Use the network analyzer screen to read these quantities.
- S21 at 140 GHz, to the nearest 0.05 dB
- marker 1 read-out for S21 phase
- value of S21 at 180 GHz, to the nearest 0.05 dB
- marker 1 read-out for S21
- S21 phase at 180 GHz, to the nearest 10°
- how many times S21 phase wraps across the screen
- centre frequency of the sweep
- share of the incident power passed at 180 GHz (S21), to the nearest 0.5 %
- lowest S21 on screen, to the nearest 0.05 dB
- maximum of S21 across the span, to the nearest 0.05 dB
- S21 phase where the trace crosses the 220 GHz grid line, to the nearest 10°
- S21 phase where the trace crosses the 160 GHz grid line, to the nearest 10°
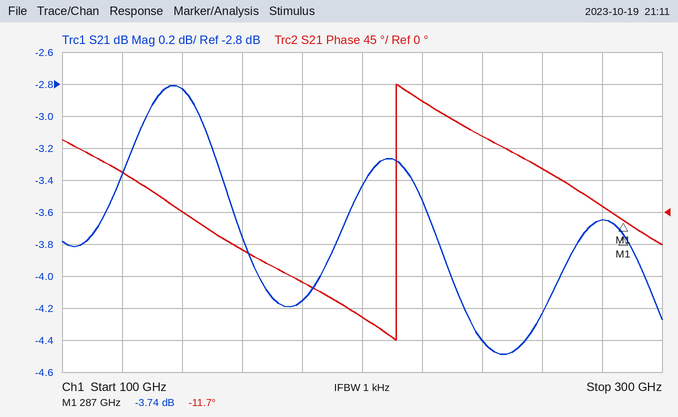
-2.85 dB
-11.7°
-4.15 dB
-3.74 dB
-100°
1
200 GHz
38.5 %
-4.50 dB
-2.80 dB
160°
-50°
